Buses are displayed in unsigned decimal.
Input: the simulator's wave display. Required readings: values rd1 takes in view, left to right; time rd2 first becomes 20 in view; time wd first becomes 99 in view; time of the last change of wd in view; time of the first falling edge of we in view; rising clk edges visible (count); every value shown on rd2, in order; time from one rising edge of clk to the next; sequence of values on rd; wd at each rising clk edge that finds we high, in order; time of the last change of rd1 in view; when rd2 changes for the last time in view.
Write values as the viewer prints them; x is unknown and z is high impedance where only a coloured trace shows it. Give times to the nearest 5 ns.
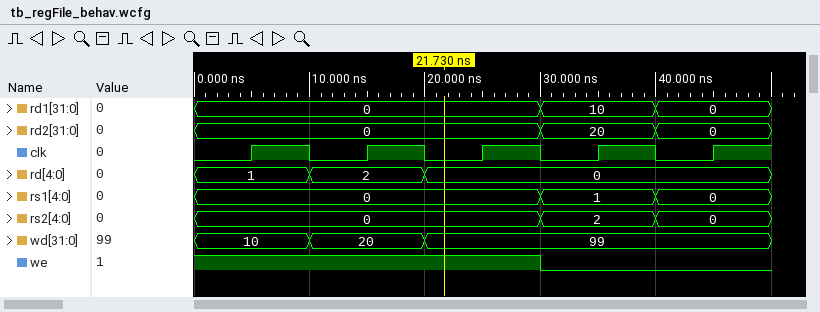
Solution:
0, 10, 0
30 ns
20 ns
20 ns
30 ns
5
0, 20, 0
10 ns
1, 2, 0
10, 20, 99
40 ns
40 ns
